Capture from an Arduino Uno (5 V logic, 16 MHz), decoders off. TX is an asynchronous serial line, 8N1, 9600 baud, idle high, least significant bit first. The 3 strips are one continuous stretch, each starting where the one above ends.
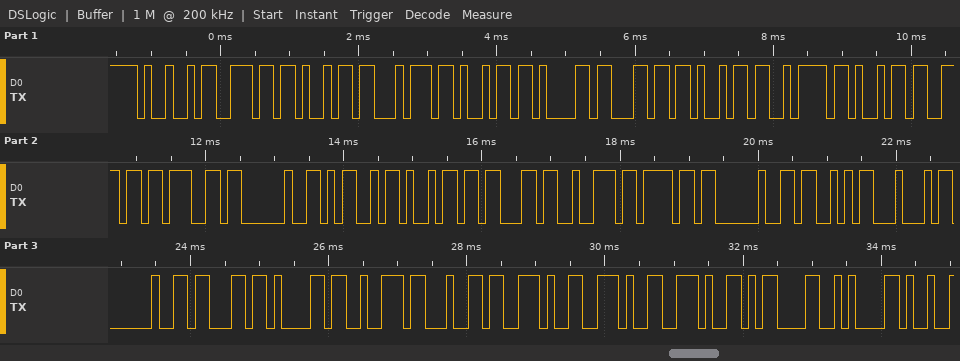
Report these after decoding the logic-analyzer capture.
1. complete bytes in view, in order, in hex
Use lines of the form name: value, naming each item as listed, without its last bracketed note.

complete bytes in view, in order, in hex: 0x49 0x6E 0x69 0x74 0x69 0x61 0x6C 0x69 0x7A 0x69 0x6E 0x67 0x20 0x4D 0x69 0x63 0x72 0x6F 0x20 0x53 0x44 0x20 0x63 0x61 0x72 0x64 0x2E 0x2E 0x2E 0x0D 0x0A
